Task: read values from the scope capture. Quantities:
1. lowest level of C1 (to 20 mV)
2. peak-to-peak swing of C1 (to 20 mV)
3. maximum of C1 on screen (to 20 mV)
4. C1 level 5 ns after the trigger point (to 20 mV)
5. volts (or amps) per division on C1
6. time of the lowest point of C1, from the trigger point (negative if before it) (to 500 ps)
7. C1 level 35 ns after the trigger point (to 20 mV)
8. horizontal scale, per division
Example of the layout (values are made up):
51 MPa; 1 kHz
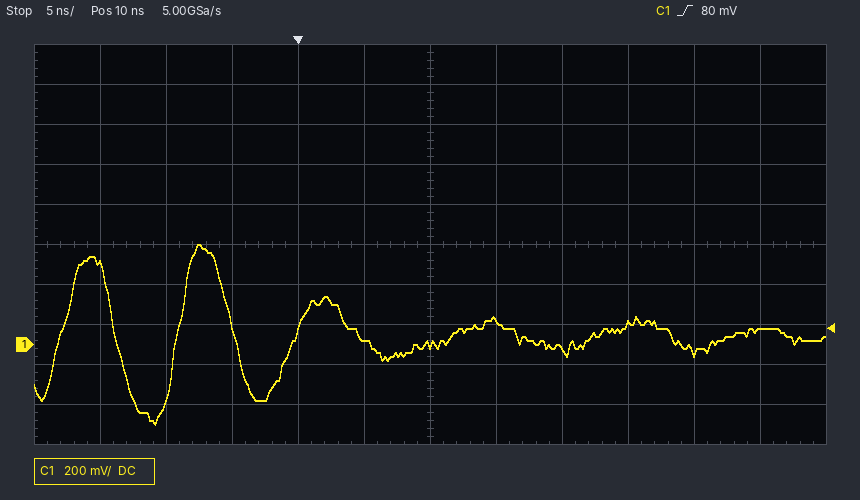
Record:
-400 mV; 900 mV; 500 mV; 20 mV; 200 mV; -11.0 ns; 80 mV; 5 ns
